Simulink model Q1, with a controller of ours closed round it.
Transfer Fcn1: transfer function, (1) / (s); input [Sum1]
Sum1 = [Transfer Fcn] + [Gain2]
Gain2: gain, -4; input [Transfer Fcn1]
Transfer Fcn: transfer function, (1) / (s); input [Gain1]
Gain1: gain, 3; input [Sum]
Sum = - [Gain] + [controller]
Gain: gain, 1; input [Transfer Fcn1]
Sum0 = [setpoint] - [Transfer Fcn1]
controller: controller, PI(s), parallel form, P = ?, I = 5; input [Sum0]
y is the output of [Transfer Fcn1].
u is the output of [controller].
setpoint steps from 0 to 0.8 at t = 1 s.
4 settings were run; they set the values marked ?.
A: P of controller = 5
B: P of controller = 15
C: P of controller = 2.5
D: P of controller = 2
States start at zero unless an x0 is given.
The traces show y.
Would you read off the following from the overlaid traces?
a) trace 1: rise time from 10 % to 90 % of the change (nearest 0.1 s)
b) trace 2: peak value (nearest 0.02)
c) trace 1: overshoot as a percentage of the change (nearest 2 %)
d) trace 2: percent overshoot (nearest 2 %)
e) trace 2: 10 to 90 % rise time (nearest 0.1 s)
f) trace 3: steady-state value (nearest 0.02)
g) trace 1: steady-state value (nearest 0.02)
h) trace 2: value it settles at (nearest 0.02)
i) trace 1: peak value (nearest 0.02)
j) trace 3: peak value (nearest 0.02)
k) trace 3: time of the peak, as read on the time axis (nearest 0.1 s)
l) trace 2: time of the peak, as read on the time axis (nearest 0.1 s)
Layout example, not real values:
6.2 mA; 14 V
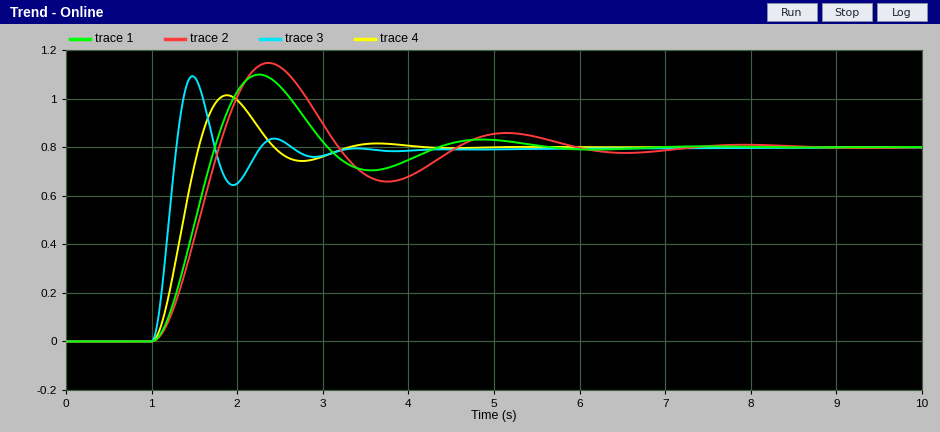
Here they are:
0.5 s; 1.14; 38 %; 44 %; 0.5 s; 0.80; 0.80; 0.80; 1.10; 1.10; 1.5 s; 2.4 s
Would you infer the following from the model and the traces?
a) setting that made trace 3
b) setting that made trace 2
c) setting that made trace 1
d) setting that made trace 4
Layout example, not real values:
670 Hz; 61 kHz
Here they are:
B; D; C; A
